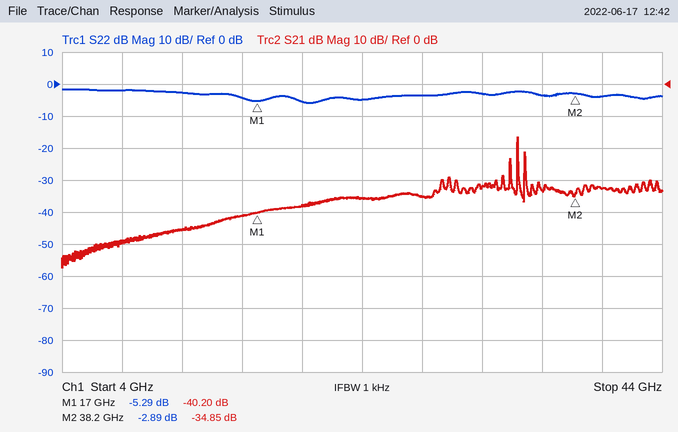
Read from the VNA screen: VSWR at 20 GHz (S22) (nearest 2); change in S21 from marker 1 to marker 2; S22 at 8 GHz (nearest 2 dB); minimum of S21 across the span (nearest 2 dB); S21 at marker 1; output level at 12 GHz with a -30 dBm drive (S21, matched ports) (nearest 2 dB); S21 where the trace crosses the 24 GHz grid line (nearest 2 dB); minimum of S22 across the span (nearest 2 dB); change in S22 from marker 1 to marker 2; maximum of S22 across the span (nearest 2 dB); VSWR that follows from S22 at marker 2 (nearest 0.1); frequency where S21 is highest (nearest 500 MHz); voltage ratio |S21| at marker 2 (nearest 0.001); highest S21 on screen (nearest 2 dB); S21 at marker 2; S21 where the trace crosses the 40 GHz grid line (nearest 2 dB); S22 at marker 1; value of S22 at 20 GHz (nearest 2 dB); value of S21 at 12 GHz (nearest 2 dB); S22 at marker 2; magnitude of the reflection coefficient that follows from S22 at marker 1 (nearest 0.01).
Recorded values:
4
5.35 dB
-2 dB
-58 dB
-40.20 dB
-76 dBm
-36 dB
-6 dB
2.40 dB
-2 dB
6.1
34.5 GHz
0.018
-16 dB
-34.85 dB
-32 dB
-5.29 dB
-6 dB
-46 dB
-2.89 dB
0.54
